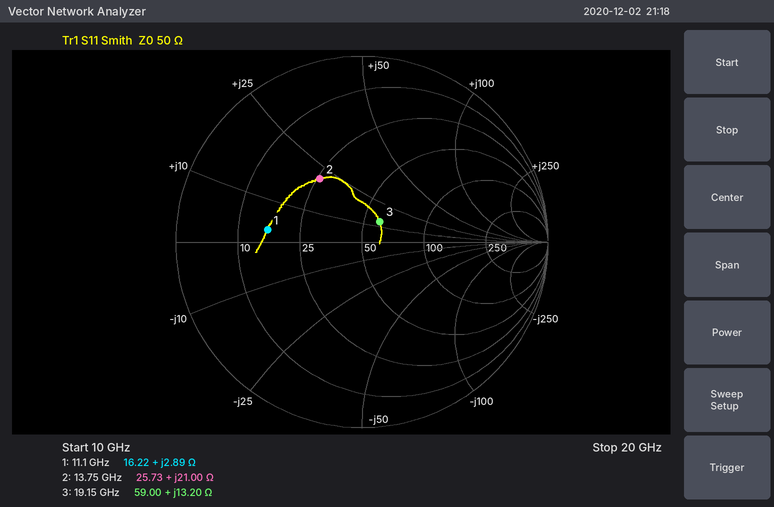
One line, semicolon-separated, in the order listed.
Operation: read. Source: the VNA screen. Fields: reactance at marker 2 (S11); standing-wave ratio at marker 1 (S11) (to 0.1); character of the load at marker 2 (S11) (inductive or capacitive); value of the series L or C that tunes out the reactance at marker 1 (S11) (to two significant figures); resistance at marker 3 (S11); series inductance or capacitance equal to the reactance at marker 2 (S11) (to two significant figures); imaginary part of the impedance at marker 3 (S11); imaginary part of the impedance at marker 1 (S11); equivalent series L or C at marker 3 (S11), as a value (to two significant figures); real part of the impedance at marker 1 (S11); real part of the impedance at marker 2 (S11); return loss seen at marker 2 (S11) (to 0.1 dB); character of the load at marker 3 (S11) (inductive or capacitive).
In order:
+21.00 Ω; 3.1; inductive; 5.0 pF; 59.00 Ω; 240 pH; +13.20 Ω; +2.89 Ω; 110 pH; 16.22 Ω; 25.73 Ω; 7.8 dB; inductive
